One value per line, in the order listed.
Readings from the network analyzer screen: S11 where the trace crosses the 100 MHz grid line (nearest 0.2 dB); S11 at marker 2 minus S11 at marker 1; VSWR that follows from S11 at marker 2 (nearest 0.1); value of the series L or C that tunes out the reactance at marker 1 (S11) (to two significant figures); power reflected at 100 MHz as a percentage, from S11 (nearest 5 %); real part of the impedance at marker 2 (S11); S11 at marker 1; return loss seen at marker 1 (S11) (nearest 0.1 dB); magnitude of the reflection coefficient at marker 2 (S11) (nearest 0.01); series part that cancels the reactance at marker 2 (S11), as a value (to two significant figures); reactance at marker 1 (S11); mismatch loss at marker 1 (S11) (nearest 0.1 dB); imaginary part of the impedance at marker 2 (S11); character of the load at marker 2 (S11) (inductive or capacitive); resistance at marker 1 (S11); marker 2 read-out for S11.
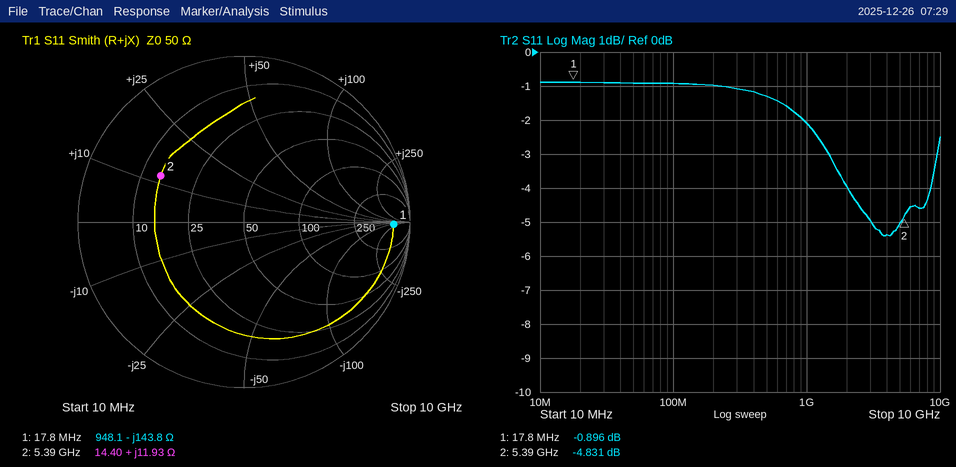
-1.0 dB
-3.935 dB
3.7
1.3 µH
80 %
14.40 Ω
-0.896 dB
0.9 dB
0.57
2.5 pF
-143.8 Ω
7.3 dB
+11.93 Ω
inductive
948.1 Ω
-4.831 dB
